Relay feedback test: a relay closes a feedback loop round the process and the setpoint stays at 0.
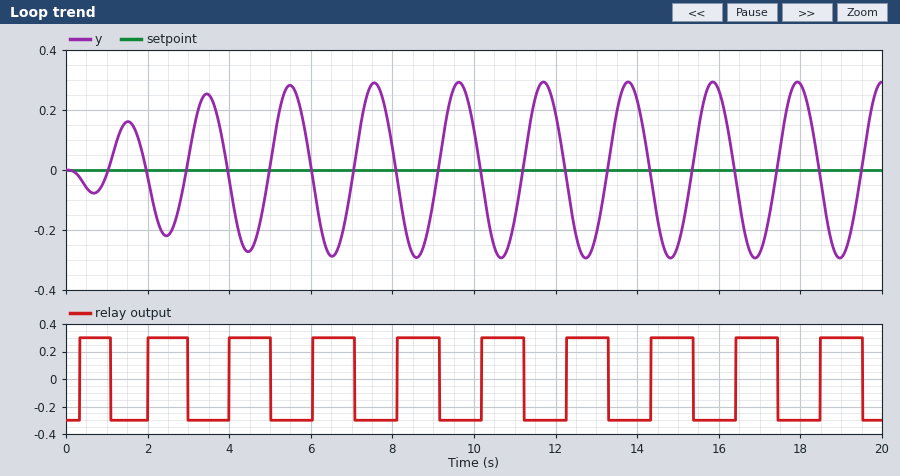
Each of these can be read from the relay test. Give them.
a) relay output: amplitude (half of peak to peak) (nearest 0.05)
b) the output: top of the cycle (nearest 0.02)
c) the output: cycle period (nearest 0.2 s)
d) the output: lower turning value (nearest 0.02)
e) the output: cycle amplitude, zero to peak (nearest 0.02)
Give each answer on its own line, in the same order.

0.30
0.30
2.0 s
-0.30
0.30
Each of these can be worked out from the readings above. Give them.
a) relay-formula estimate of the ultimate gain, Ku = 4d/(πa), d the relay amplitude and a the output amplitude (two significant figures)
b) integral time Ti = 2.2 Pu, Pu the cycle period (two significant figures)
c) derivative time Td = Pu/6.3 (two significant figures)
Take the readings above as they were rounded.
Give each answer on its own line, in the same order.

1.3
4.4 s
0.32 s
